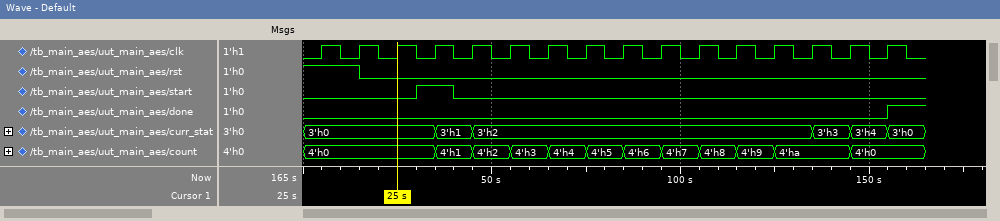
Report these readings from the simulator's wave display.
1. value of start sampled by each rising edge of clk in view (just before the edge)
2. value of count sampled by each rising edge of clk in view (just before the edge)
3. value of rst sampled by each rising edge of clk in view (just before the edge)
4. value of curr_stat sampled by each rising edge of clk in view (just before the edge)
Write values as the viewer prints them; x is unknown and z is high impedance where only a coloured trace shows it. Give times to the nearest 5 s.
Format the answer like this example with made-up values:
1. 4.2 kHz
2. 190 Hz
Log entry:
1. 0 0 0 1 0 0 0 0 0 0 0 0 0 0 0 0
2. 4'h0, 4'h0, 4'h0, 4'h0, 4'h1, 4'h2, 4'h3, 4'h4, 4'h5, 4'h6, 4'h7, 4'h8, 4'h9, 4'ha, 4'ha, 4'h0
3. 1 1 0 0 0 0 0 0 0 0 0 0 0 0 0 0
4. 3'h0, 3'h0, 3'h0, 3'h0, 3'h1, 3'h2, 3'h2, 3'h2, 3'h2, 3'h2, 3'h2, 3'h2, 3'h2, 3'h2, 3'h3, 3'h4
